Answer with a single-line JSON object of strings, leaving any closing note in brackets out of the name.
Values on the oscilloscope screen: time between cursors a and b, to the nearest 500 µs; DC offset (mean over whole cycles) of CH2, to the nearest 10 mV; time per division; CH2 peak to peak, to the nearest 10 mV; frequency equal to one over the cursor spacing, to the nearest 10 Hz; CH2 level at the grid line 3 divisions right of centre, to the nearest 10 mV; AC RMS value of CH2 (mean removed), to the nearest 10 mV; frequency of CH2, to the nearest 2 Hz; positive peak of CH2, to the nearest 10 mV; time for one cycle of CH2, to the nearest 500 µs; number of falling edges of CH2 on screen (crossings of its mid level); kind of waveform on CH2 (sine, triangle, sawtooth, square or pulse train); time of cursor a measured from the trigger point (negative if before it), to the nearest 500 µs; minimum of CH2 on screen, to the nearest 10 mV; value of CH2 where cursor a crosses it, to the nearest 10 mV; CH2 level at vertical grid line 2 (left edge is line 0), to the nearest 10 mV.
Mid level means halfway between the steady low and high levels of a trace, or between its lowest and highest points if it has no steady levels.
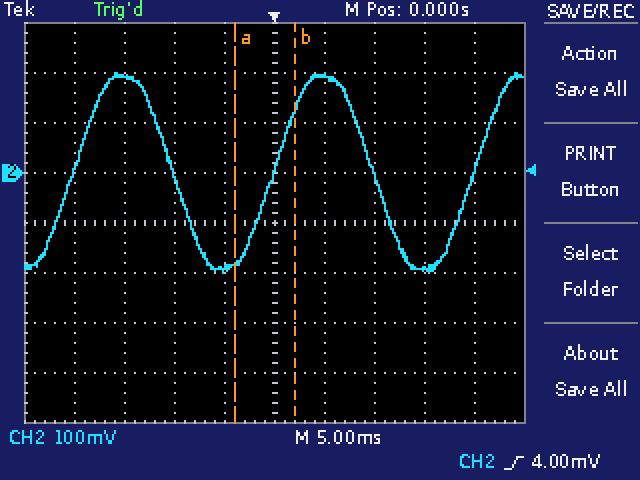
{"time between cursors a and b, to the nearest 500 µs": "6.0 ms", "DC offset (mean over whole cycles) of CH2, to the nearest 10 mV": "0 mV", "time per division": "5 ms", "CH2 peak to peak, to the nearest 10 mV": "400 mV", "frequency equal to one over the cursor spacing, to the nearest 10 Hz": "170 Hz", "CH2 level at the grid line 3 divisions right of centre, to the nearest 10 mV": "-190 mV", "AC RMS value of CH2 (mean removed), to the nearest 10 mV": "140 mV", "frequency of CH2, to the nearest 2 Hz": "50 Hz", "positive peak of CH2, to the nearest 10 mV": "200 mV", "time for one cycle of CH2, to the nearest 500 µs": "20.0 ms", "number of falling edges of CH2 on screen": "2", "kind of waveform on CH2": "sine", "time of cursor a measured from the trigger point (negative if before it), to the nearest 500 µs": "-4.0 ms", "minimum of CH2 on screen, to the nearest 10 mV": "-200 mV", "value of CH2 where cursor a crosses it, to the nearest 10 mV": "-180 mV", "CH2 level at vertical grid line 2 (left edge is line 0), to the nearest 10 mV": "190 mV"}
